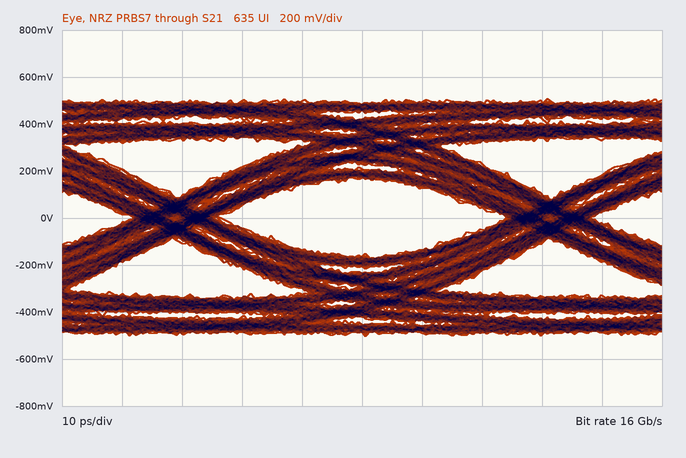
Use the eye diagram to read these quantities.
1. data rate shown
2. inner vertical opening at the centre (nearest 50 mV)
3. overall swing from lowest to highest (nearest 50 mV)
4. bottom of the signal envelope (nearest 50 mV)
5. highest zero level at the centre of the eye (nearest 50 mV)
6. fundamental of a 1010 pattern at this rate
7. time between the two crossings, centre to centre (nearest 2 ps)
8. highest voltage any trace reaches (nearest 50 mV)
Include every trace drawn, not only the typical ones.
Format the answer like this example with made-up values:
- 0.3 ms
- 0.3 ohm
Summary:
- 16 Gb/s
- 350 mV
- 1.00 V
- -500 mV
- -150 mV
- 8 GHz
- 62 ps
- 500 mV
